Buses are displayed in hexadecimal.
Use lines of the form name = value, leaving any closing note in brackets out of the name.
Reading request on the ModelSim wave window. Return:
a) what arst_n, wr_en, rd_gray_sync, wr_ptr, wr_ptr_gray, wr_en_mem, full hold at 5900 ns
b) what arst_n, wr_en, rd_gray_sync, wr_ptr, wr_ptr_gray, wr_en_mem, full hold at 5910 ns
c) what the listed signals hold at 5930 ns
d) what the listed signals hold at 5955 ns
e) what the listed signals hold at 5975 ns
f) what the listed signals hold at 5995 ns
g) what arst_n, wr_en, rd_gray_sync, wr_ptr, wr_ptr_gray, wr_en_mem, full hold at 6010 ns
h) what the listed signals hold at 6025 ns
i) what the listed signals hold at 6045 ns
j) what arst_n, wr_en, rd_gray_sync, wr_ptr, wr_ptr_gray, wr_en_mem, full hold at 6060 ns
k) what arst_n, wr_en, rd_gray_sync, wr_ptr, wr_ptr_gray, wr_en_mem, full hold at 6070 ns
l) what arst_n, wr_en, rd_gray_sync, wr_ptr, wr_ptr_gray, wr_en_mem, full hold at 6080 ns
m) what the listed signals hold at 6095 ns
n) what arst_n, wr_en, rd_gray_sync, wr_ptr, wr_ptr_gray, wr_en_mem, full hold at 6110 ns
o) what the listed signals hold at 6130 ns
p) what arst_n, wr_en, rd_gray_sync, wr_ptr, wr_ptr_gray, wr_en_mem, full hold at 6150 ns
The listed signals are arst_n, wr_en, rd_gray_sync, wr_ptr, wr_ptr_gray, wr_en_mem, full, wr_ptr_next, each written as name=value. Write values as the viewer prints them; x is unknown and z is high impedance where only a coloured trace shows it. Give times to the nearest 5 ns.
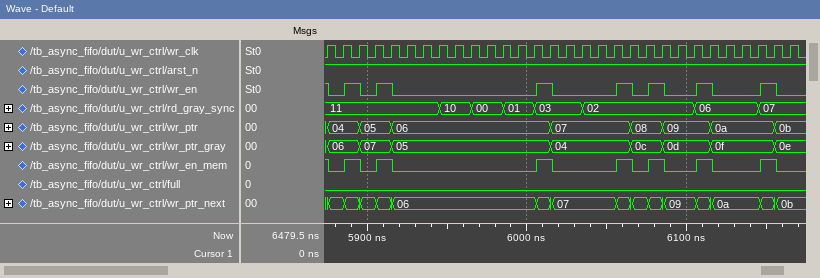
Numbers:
what arst_n, wr_en, rd_gray_sync, wr_ptr, wr_ptr_gray, wr_en_mem, full hold at 5900 ns = arst_n=1, wr_en=0, rd_gray_sync=11, wr_ptr=05, wr_ptr_gray=07, wr_en_mem=0, full=0
what arst_n, wr_en, rd_gray_sync, wr_ptr, wr_ptr_gray, wr_en_mem, full hold at 5910 ns = arst_n=1, wr_en=1, rd_gray_sync=11, wr_ptr=05, wr_ptr_gray=07, wr_en_mem=1, full=0
what the listed signals hold at 5930 ns = arst_n=1, wr_en=0, rd_gray_sync=11, wr_ptr=06, wr_ptr_gray=05, wr_en_mem=0, full=0, wr_ptr_next=06
what the listed signals hold at 5955 ns = arst_n=1, wr_en=0, rd_gray_sync=10, wr_ptr=06, wr_ptr_gray=05, wr_en_mem=0, full=0, wr_ptr_next=06
what the listed signals hold at 5975 ns = arst_n=1, wr_en=0, rd_gray_sync=00, wr_ptr=06, wr_ptr_gray=05, wr_en_mem=0, full=0, wr_ptr_next=06
what the listed signals hold at 5995 ns = arst_n=1, wr_en=0, rd_gray_sync=01, wr_ptr=06, wr_ptr_gray=05, wr_en_mem=0, full=0, wr_ptr_next=06
what arst_n, wr_en, rd_gray_sync, wr_ptr, wr_ptr_gray, wr_en_mem, full hold at 6010 ns = arst_n=1, wr_en=1, rd_gray_sync=03, wr_ptr=06, wr_ptr_gray=05, wr_en_mem=1, full=0
what the listed signals hold at 6025 ns = arst_n=1, wr_en=0, rd_gray_sync=03, wr_ptr=07, wr_ptr_gray=04, wr_en_mem=0, full=0, wr_ptr_next=07
what the listed signals hold at 6045 ns = arst_n=1, wr_en=0, rd_gray_sync=02, wr_ptr=07, wr_ptr_gray=04, wr_en_mem=0, full=0, wr_ptr_next=07
what arst_n, wr_en, rd_gray_sync, wr_ptr, wr_ptr_gray, wr_en_mem, full hold at 6060 ns = arst_n=1, wr_en=1, rd_gray_sync=02, wr_ptr=07, wr_ptr_gray=04, wr_en_mem=1, full=0
what arst_n, wr_en, rd_gray_sync, wr_ptr, wr_ptr_gray, wr_en_mem, full hold at 6070 ns = arst_n=1, wr_en=0, rd_gray_sync=02, wr_ptr=08, wr_ptr_gray=0c, wr_en_mem=0, full=0
what arst_n, wr_en, rd_gray_sync, wr_ptr, wr_ptr_gray, wr_en_mem, full hold at 6080 ns = arst_n=1, wr_en=1, rd_gray_sync=02, wr_ptr=08, wr_ptr_gray=0c, wr_en_mem=1, full=0
what the listed signals hold at 6095 ns = arst_n=1, wr_en=0, rd_gray_sync=02, wr_ptr=09, wr_ptr_gray=0d, wr_en_mem=0, full=0, wr_ptr_next=09
what arst_n, wr_en, rd_gray_sync, wr_ptr, wr_ptr_gray, wr_en_mem, full hold at 6110 ns = arst_n=1, wr_en=1, rd_gray_sync=06, wr_ptr=09, wr_ptr_gray=0d, wr_en_mem=1, full=0
what the listed signals hold at 6130 ns = arst_n=1, wr_en=0, rd_gray_sync=06, wr_ptr=0a, wr_ptr_gray=0f, wr_en_mem=0, full=0, wr_ptr_next=0a
what arst_n, wr_en, rd_gray_sync, wr_ptr, wr_ptr_gray, wr_en_mem, full hold at 6150 ns = arst_n=1, wr_en=1, rd_gray_sync=07, wr_ptr=0a, wr_ptr_gray=0f, wr_en_mem=1, full=0
